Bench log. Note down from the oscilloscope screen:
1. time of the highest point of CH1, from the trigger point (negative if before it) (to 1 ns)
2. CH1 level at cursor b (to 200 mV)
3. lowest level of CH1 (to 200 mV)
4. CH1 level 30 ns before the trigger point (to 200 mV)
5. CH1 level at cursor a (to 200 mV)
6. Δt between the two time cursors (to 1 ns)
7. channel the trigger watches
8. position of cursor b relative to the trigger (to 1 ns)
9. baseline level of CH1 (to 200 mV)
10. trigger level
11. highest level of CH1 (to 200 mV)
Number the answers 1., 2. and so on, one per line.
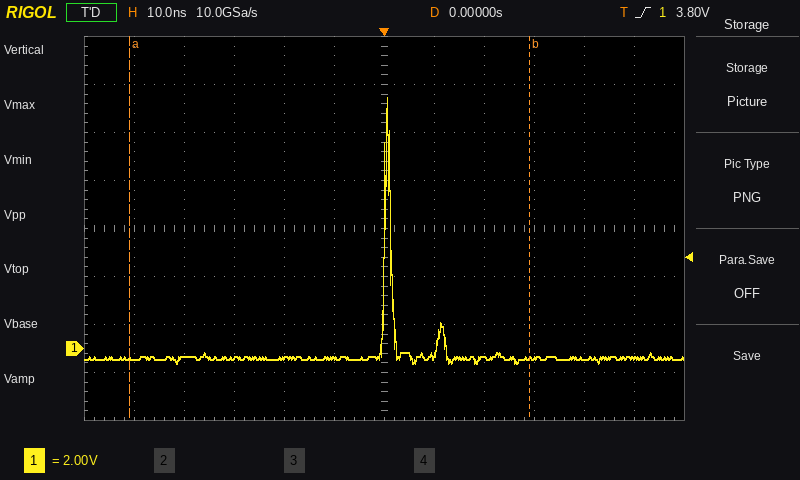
1. +1 ns
2. -400 mV
3. -600 mV
4. -400 mV
5. -400 mV
6. 80 ns
7. CH1
8. +29 ns
9. -400 mV
10. 3.80 V
11. 10.4 V
